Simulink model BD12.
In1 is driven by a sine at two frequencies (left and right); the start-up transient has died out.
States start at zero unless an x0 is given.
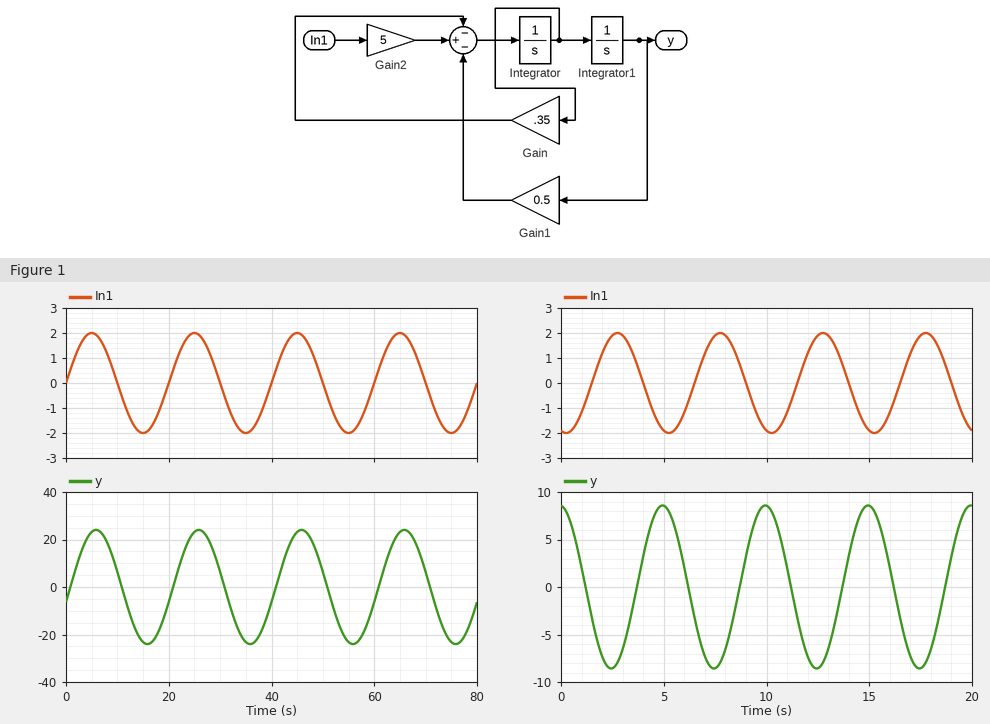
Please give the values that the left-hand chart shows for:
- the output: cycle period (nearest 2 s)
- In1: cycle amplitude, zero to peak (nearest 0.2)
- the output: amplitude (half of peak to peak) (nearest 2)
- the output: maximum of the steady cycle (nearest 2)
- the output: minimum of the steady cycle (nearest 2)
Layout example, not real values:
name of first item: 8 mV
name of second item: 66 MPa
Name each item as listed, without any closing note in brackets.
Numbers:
the output: cycle period: 20 s
In1: cycle amplitude, zero to peak: 2.0
the output: amplitude (half of peak to peak): 24
the output: maximum of the steady cycle: 24
the output: minimum of the steady cycle: -24
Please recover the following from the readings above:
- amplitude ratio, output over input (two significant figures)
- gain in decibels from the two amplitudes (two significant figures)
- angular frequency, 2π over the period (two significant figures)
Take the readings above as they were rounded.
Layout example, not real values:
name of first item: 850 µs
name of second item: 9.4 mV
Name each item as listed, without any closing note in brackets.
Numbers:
amplitude ratio, output over input: 12
gain in decibels from the two amplitudes: 22 dB
angular frequency, 2π over the period: 0.31 rad/s
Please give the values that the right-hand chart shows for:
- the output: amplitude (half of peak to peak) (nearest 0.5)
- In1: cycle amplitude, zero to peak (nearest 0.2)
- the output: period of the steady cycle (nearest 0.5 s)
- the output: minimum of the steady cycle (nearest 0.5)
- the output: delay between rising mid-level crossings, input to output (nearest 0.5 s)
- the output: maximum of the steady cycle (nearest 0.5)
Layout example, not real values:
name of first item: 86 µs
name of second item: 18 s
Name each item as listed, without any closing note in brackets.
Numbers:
the output: amplitude (half of peak to peak): 8.5
In1: cycle amplitude, zero to peak: 2.0
the output: period of the steady cycle: 5.0 s
the output: minimum of the steady cycle: -8.5
the output: delay between rising mid-level crossings, input to output: 2.0 s
the output: maximum of the steady cycle: 8.5
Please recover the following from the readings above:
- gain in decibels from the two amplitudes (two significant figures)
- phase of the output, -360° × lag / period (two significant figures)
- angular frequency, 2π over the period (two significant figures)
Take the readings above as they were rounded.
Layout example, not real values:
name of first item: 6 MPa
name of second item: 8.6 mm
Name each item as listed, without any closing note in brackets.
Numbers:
gain in decibels from the two amplitudes: 13 dB
phase of the output, -360° × lag / period: -140°
angular frequency, 2π over the period: 1.3 rad/s
